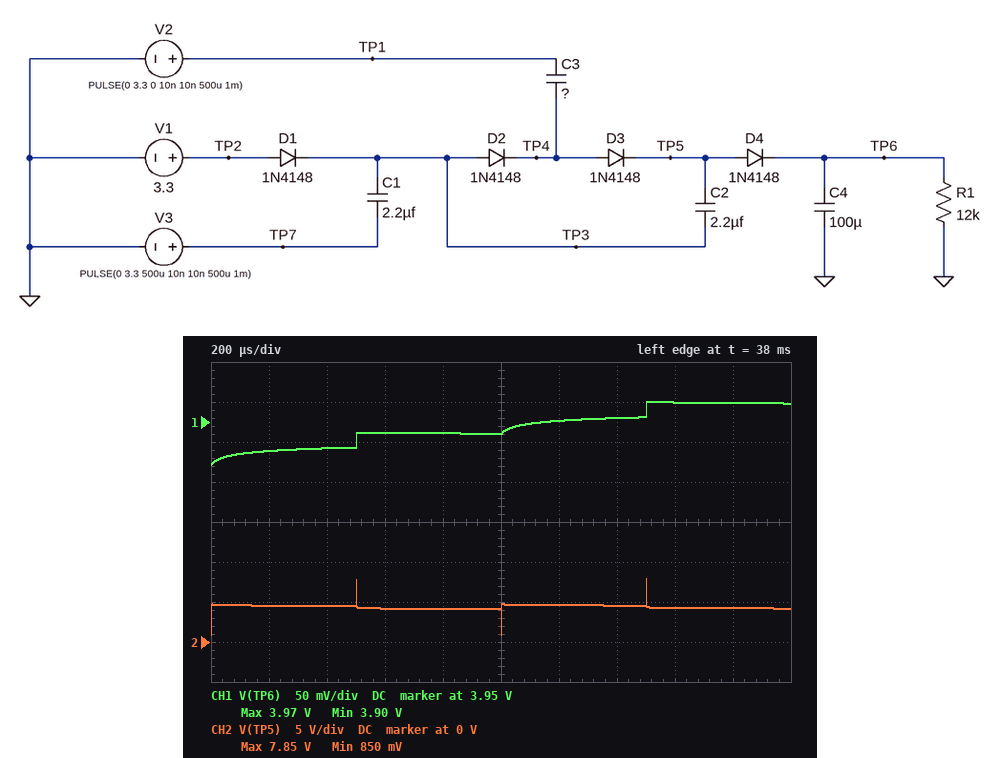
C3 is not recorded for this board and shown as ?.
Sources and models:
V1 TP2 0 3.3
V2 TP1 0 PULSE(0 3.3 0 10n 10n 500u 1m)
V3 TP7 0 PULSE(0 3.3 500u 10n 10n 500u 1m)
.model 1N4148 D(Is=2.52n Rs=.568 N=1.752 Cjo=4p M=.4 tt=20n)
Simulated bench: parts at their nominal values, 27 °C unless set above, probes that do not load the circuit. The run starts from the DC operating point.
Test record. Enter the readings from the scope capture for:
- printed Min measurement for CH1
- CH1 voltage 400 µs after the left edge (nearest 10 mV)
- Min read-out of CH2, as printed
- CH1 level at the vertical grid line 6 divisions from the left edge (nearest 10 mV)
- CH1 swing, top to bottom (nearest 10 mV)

3.90 V
3.92 V
850 mV
3.95 V
80 mV
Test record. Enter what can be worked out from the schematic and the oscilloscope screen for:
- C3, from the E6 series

4.7 µF
